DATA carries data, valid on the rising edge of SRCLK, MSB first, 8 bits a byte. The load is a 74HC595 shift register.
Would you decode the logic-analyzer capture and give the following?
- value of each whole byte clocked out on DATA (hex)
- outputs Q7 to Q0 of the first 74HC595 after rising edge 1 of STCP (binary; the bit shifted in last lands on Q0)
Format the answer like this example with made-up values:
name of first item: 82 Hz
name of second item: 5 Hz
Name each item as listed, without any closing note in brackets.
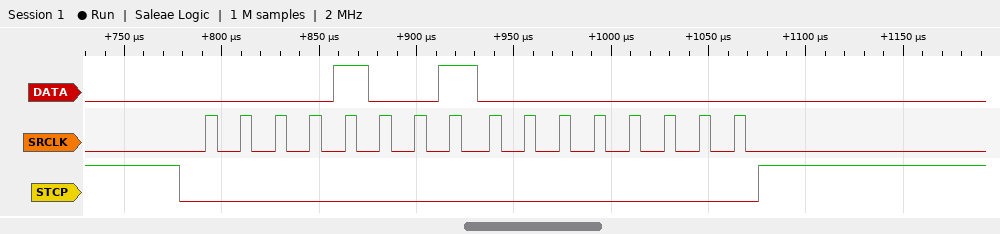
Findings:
value of each whole byte clocked out on DATA: 09 00
outputs Q7 to Q0 of the first 74HC595 after rising edge 1 of STCP: 00000000
